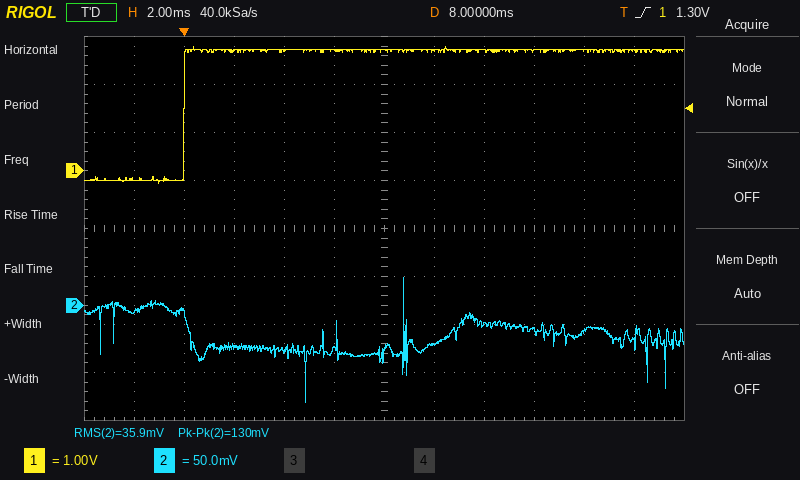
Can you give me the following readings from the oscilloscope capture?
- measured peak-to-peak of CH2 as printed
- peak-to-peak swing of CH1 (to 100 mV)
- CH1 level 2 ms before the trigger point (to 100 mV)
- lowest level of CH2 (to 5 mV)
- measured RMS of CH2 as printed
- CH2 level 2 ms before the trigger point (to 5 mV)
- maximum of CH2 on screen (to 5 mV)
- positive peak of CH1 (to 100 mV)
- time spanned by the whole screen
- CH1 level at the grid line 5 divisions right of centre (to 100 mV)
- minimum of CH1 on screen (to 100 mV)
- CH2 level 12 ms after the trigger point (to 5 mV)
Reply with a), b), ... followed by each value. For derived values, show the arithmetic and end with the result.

a) 130 mV
b) 2.6 V − (-300 mV) = 2.9 V
c) -200 mV
d) -100 mV
e) 35.9 mV
f) -5 mV
g) 30 mV
h) 2.6 V
i) 24 ms
j) 2.5 V
k) -300 mV
l) -20 mV
